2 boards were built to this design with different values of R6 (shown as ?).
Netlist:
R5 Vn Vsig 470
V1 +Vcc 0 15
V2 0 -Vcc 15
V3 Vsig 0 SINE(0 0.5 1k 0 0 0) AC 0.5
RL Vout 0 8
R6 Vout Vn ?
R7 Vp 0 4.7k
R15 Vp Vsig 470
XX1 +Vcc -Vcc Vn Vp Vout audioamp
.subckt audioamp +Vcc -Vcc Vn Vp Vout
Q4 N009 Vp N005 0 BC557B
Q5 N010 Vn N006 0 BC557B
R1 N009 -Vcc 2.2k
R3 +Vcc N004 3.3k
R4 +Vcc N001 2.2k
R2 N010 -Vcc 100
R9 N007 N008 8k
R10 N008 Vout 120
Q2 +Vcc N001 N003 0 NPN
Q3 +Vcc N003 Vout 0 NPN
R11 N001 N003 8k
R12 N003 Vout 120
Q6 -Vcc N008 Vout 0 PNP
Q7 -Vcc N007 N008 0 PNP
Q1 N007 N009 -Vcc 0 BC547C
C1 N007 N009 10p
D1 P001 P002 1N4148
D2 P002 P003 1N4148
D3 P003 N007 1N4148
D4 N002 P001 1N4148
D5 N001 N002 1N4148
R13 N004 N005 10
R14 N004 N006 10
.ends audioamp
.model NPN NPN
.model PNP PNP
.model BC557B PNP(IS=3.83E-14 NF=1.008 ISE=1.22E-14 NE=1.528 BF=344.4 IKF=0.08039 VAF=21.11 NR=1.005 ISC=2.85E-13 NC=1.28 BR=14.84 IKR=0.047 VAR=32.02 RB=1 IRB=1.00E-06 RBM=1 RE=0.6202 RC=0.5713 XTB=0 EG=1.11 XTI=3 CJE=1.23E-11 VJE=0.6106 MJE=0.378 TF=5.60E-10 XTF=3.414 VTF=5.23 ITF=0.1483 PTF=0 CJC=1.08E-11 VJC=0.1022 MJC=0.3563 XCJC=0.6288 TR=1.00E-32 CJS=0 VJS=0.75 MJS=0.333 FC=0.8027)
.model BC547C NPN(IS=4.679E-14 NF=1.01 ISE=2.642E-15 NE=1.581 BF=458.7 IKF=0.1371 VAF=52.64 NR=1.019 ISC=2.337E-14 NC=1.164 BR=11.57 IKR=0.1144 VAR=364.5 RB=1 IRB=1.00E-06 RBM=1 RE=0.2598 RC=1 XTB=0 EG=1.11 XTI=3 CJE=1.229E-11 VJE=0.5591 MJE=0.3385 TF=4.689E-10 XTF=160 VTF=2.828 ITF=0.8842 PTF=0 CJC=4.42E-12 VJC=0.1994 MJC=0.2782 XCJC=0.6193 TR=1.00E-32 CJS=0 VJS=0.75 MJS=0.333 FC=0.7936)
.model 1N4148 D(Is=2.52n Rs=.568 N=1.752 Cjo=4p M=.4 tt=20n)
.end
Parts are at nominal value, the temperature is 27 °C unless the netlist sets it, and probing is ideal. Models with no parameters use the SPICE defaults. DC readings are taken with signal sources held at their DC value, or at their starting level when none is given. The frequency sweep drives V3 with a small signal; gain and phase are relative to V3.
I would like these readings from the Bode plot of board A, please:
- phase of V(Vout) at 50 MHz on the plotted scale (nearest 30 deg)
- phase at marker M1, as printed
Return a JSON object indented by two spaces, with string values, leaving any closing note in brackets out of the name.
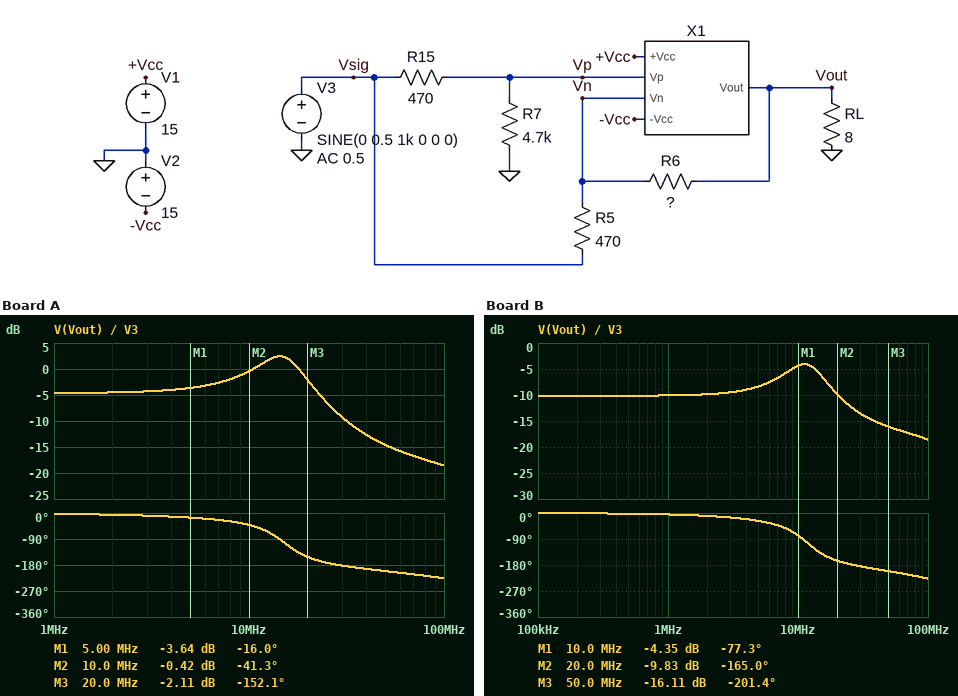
{
  "phase of V(Vout) at 50 MHz on the plotted scale": "-210 deg",
  "phase at marker M1, as printed": "-16.0 deg"
}
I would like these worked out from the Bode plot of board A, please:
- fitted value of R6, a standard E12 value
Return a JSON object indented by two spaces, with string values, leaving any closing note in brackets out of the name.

{
  "fitted value of R6, a standard E12 value": "1.8 kΩ"
}
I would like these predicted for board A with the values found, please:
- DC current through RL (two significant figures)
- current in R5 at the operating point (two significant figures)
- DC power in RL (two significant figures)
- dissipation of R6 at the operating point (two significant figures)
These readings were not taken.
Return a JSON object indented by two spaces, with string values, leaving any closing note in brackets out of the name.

{
  "DC current through RL": "66 mA",
  "current in R5 at the operating point": "230 µA",
  "DC power in RL": "35 mW",
  "dissipation of R6 at the operating point": "99 µW"
}
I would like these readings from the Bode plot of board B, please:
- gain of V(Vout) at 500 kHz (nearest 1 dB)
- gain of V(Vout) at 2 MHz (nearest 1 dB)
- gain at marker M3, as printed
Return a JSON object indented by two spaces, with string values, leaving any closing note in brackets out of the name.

{
  "gain of V(Vout) at 500 kHz": "-10 dB",
  "gain of V(Vout) at 2 MHz": "-10 dB",
  "gain at marker M3, as printed": "-16.11 dB"
}
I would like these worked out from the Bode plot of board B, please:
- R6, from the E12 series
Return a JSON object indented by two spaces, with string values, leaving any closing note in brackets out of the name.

{
  "R6, from the E12 series": "3.3 kΩ"
}
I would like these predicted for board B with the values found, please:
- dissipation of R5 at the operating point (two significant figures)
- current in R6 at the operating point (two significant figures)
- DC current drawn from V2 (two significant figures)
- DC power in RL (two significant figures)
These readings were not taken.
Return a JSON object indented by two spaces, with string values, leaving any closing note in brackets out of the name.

{
  "dissipation of R5 at the operating point": "24 µW",
  "current in R6 at the operating point": "230 µA",
  "DC current drawn from V2": "130 mA",
  "DC power in RL": "97 mW"
}
